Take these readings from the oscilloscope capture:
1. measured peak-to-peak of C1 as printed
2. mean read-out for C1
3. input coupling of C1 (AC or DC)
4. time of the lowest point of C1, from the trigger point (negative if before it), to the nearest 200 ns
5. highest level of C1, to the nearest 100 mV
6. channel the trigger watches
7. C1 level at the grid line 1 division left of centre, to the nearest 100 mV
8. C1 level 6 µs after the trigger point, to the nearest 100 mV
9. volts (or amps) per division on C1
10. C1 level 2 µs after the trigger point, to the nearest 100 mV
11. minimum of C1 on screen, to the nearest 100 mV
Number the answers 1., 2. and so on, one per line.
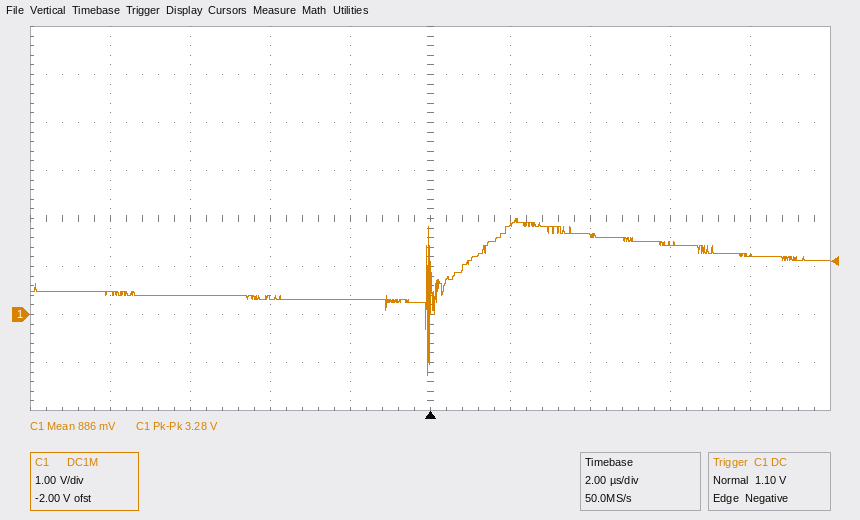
1. 3.28 V
2. 886 mV
3. DC
4. 0.0 µs
5. 2.0 V
6. C1
7. 300 mV
8. 1.5 V
9. 1 V
10. 1.9 V
11. -1.3 V
